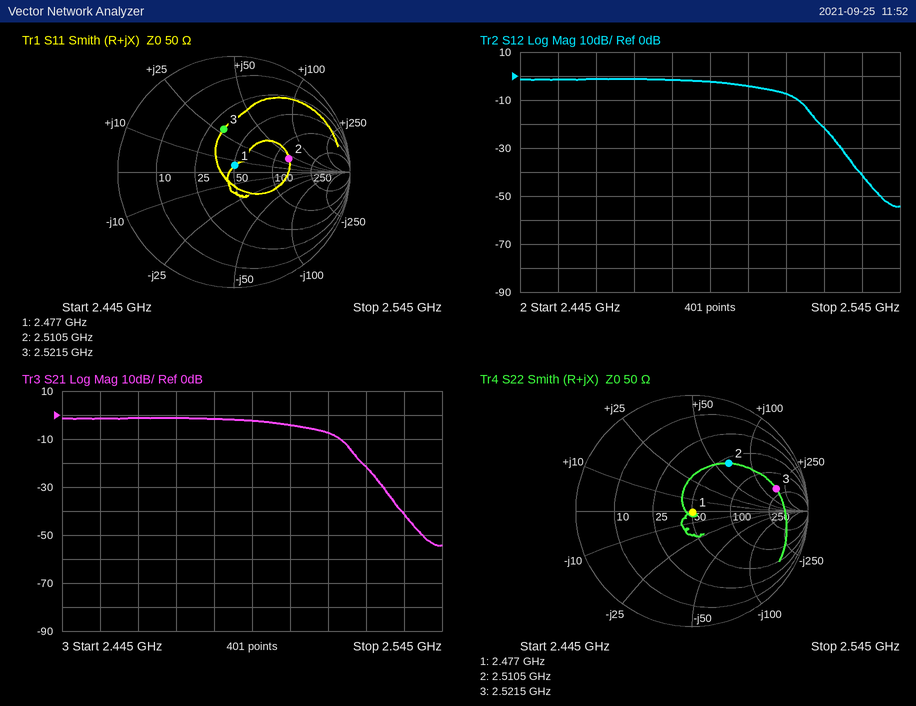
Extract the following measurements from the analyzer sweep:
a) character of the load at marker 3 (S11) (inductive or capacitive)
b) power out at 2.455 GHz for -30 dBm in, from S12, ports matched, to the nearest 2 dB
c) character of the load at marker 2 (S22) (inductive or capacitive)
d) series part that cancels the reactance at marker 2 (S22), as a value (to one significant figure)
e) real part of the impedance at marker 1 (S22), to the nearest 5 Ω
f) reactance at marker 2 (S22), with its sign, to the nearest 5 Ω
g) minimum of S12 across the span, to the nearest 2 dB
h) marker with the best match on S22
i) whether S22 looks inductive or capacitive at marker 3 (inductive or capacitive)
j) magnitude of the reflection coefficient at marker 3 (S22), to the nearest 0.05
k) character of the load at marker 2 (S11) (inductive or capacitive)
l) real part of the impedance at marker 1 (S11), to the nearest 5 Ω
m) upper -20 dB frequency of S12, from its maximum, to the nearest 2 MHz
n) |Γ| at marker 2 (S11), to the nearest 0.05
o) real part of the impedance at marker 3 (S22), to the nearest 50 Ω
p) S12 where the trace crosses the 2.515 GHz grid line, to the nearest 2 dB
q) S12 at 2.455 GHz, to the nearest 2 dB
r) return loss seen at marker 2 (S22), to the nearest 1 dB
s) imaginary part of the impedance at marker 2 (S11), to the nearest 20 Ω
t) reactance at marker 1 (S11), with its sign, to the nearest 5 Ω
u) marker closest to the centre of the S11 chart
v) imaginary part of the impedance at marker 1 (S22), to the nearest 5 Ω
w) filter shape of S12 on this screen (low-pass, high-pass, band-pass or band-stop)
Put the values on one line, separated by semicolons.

inductive; -32 dBm; inductive; 1.0 pF; 50 Ω; +65 Ω; -54 dB; marker 1; inductive; 0.75; inductive; 50 Ω; 2.524 GHz; 0.50; 200 Ω; -8 dB; -2 dB; 6 dB; +40 Ω; +5 Ω; marker 1; 0 Ω; low-pass
